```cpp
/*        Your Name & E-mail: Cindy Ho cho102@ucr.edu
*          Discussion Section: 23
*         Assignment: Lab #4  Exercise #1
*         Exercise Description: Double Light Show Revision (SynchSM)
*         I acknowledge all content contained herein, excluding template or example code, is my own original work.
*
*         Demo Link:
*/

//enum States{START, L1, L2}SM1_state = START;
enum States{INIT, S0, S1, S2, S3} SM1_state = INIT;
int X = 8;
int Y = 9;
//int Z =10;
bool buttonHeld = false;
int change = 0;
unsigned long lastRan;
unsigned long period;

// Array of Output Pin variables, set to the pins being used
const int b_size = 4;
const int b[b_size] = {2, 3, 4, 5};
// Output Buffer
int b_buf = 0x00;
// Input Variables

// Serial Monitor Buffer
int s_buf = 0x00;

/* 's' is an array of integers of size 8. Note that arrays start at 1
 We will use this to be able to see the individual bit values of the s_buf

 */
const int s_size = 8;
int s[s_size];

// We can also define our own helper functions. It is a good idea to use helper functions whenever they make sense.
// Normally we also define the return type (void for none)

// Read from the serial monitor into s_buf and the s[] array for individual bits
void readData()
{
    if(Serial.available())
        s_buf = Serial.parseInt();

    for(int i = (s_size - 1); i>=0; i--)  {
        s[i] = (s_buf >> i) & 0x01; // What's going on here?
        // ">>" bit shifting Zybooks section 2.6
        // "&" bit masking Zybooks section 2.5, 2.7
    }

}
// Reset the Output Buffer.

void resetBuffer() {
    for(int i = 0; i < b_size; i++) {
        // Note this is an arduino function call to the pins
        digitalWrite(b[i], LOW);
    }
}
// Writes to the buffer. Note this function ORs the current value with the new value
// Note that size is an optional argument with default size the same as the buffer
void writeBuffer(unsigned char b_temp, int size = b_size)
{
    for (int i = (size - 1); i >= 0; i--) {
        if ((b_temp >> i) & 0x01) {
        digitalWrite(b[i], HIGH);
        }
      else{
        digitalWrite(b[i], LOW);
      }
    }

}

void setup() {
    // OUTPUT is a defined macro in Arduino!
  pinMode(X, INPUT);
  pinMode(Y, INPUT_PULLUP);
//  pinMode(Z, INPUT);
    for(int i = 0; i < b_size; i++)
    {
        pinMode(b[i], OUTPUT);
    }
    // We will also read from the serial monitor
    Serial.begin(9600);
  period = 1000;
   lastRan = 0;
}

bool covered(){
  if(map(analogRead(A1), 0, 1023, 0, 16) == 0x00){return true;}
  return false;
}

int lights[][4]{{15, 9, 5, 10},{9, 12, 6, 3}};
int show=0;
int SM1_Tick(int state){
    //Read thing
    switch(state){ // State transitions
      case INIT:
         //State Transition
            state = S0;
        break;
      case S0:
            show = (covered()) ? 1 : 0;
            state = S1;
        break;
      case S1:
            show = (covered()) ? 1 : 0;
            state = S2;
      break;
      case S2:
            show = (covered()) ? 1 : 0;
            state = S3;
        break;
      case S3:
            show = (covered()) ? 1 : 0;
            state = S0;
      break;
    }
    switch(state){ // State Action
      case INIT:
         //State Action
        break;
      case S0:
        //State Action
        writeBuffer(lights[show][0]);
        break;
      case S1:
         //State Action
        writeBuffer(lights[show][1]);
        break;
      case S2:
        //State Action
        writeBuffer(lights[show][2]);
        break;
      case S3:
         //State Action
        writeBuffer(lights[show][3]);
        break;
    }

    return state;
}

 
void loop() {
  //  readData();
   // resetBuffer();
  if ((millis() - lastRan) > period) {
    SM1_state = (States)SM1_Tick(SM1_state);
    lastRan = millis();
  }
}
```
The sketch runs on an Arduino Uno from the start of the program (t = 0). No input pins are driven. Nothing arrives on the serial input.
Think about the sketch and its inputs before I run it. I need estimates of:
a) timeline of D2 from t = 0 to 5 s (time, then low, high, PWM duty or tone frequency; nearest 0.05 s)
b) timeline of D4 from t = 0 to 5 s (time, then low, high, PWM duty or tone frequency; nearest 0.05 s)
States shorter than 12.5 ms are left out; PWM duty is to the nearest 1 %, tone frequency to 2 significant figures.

0 s low; 1 s high; 2 s low; 4 s high
0 s low; 1 s high; 4 s low
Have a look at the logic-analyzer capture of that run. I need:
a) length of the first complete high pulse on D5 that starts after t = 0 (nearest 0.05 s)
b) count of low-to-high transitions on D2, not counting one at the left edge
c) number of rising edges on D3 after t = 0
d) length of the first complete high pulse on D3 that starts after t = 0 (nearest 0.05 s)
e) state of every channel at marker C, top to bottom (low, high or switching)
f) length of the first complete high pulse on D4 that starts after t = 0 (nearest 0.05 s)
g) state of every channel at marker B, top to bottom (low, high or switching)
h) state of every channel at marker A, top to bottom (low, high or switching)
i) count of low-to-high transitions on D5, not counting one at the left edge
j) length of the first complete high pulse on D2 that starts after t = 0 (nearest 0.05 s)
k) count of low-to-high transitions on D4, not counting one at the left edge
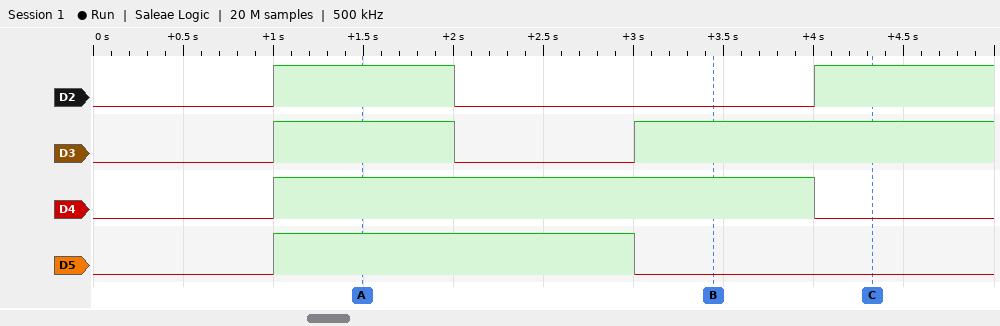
2.00 s
2
2
1.00 s
D2 high, D3 high, D4 low, D5 low
3.00 s
D2 low, D3 high, D4 high, D5 low
D2 high, D3 high, D4 high, D5 high
1
1.00 s
1
